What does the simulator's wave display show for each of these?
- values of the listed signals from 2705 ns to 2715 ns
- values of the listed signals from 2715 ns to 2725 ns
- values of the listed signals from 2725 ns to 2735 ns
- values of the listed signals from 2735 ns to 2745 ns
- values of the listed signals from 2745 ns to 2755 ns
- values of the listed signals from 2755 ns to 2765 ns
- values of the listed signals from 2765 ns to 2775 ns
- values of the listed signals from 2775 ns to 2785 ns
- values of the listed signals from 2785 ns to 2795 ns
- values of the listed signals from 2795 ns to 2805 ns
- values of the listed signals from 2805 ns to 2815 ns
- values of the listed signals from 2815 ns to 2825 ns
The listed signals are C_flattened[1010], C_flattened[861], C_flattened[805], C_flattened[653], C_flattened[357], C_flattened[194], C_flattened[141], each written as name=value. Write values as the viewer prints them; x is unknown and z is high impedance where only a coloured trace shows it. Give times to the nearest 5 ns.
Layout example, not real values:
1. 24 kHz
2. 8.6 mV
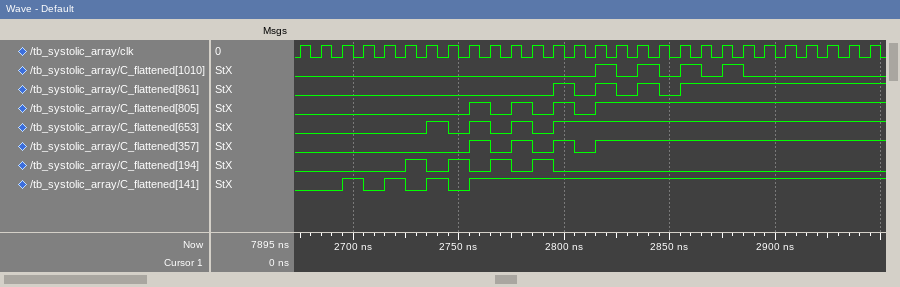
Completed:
1. C_flattened[1010]=0, C_flattened[861]=0, C_flattened[805]=0, C_flattened[653]=0, C_flattened[357]=0, C_flattened[194]=0, C_flattened[141]=0
2. C_flattened[1010]=0, C_flattened[861]=0, C_flattened[805]=0, C_flattened[653]=0, C_flattened[357]=0, C_flattened[194]=0, C_flattened[141]=1
3. C_flattened[1010]=0, C_flattened[861]=0, C_flattened[805]=0, C_flattened[653]=0, C_flattened[357]=0, C_flattened[194]=1, C_flattened[141]=0
4. C_flattened[1010]=0, C_flattened[861]=0, C_flattened[805]=0, C_flattened[653]=1, C_flattened[357]=0, C_flattened[194]=0, C_flattened[141]=1
5. C_flattened[1010]=0, C_flattened[861]=0, C_flattened[805]=0, C_flattened[653]=0, C_flattened[357]=0, C_flattened[194]=1, C_flattened[141]=0
6. C_flattened[1010]=0, C_flattened[861]=0, C_flattened[805]=1, C_flattened[653]=1, C_flattened[357]=1, C_flattened[194]=0, C_flattened[141]=1
7. C_flattened[1010]=0, C_flattened[861]=0, C_flattened[805]=0, C_flattened[653]=0, C_flattened[357]=0, C_flattened[194]=1, C_flattened[141]=1
8. C_flattened[1010]=0, C_flattened[861]=0, C_flattened[805]=1, C_flattened[653]=1, C_flattened[357]=1, C_flattened[194]=0, C_flattened[141]=1
9. C_flattened[1010]=0, C_flattened[861]=0, C_flattened[805]=0, C_flattened[653]=0, C_flattened[357]=0, C_flattened[194]=1, C_flattened[141]=1
10. C_flattened[1010]=0, C_flattened[861]=1, C_flattened[805]=1, C_flattened[653]=1, C_flattened[357]=1, C_flattened[194]=0, C_flattened[141]=1
11. C_flattened[1010]=0, C_flattened[861]=0, C_flattened[805]=0, C_flattened[653]=1, C_flattened[357]=0, C_flattened[194]=0, C_flattened[141]=1
12. C_flattened[1010]=1, C_flattened[861]=1, C_flattened[805]=1, C_flattened[653]=1, C_flattened[357]=1, C_flattened[194]=0, C_flattened[141]=1
